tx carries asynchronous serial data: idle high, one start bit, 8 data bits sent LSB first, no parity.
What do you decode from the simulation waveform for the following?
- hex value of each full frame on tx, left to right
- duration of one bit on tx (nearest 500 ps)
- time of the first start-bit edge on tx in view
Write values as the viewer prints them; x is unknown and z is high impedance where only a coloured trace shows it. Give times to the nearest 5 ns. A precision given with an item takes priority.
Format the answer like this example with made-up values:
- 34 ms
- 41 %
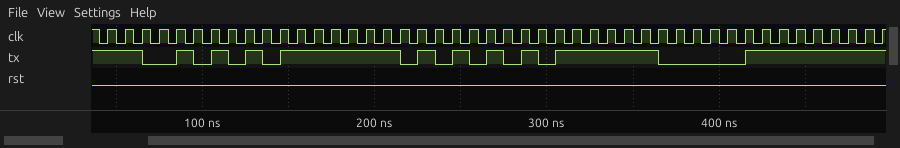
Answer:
- AA, 55, F0
- 10000 ps
- 65 ns
